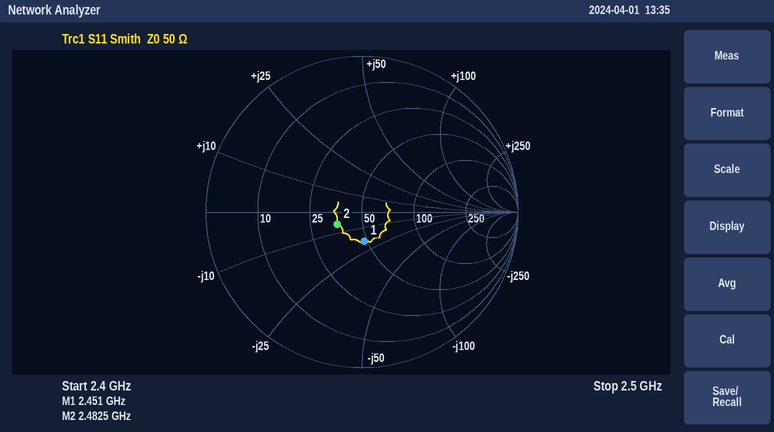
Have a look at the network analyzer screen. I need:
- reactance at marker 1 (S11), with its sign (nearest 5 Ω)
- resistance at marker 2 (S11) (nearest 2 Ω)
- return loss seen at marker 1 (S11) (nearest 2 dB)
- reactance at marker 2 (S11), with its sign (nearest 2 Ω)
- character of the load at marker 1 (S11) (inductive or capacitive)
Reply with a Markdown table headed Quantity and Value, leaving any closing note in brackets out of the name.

| Quantity | Value |
|---|---|
| reactance at marker 1 (S11), with its sign | -20 Ω |
| resistance at marker 2 (S11) | 36 Ω |
| return loss seen at marker 1 (S11) | 14 dB |
| reactance at marker 2 (S11), with its sign | -6 Ω |
| character of the load at marker 1 (S11) | capacitive |
